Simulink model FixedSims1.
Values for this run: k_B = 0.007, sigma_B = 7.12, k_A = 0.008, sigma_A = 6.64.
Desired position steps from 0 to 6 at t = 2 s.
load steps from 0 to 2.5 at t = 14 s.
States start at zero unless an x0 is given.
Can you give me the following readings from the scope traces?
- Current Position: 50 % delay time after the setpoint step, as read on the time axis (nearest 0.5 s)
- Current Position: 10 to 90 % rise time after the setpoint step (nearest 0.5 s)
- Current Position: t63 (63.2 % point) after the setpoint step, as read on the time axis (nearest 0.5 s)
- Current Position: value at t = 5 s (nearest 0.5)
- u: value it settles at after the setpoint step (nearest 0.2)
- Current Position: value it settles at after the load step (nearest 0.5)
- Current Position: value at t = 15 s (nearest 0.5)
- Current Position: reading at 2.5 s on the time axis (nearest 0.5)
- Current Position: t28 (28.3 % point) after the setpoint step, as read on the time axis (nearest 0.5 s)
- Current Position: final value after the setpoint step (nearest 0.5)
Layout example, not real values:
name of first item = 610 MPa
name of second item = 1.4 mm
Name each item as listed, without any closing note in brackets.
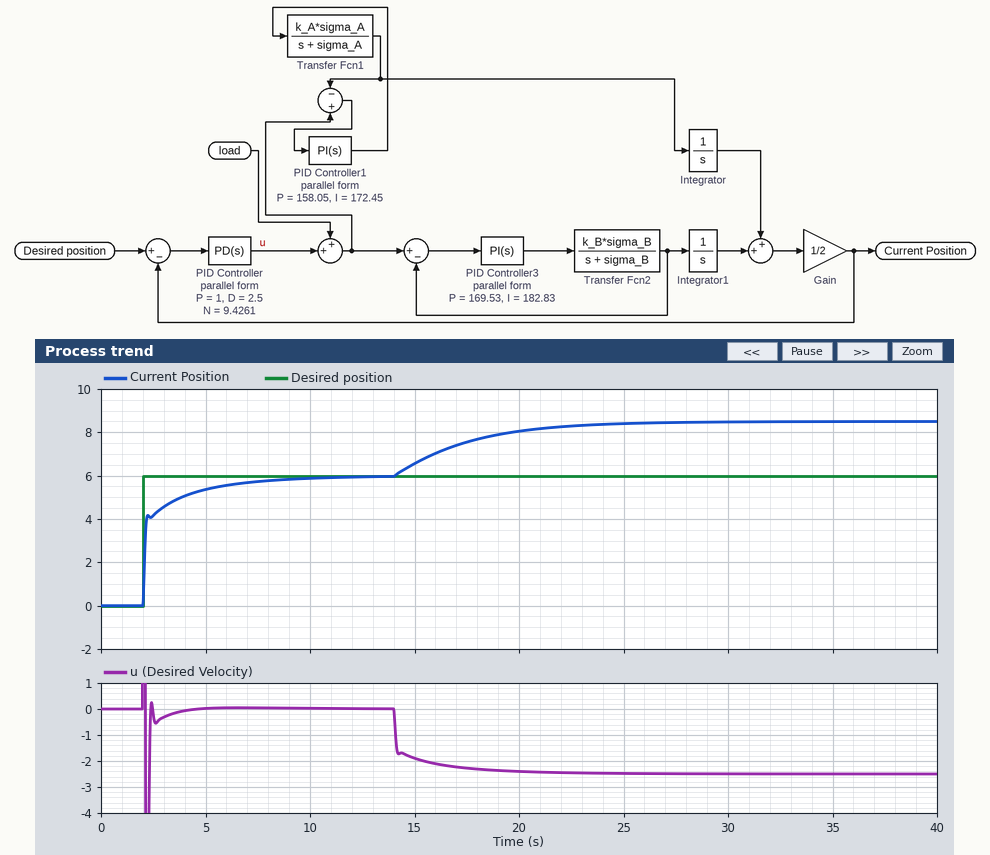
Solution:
Current Position: 50 % delay time after the setpoint step, as read on the time axis = 2.0 s
Current Position: 10 to 90 % rise time after the setpoint step = 3.0 s
Current Position: t63 (63.2 % point) after the setpoint step, as read on the time axis = 2.0 s
Current Position: value at t = 5 s = 5.5
u: value it settles at after the setpoint step = 0.0
Current Position: value it settles at after the load step = 8.5
Current Position: value at t = 15 s = 6.5
Current Position: reading at 2.5 s on the time axis = 4.0
Current Position: t28 (28.3 % point) after the setpoint step, as read on the time axis = 2.0 s
Current Position: final value after the setpoint step = 6.0
